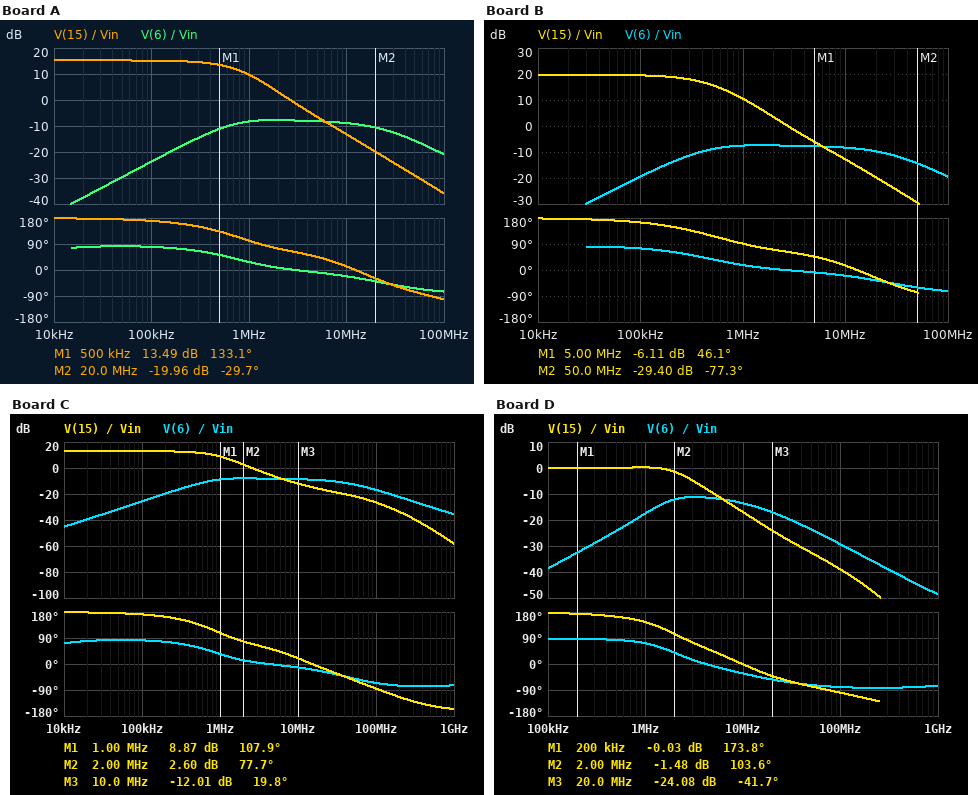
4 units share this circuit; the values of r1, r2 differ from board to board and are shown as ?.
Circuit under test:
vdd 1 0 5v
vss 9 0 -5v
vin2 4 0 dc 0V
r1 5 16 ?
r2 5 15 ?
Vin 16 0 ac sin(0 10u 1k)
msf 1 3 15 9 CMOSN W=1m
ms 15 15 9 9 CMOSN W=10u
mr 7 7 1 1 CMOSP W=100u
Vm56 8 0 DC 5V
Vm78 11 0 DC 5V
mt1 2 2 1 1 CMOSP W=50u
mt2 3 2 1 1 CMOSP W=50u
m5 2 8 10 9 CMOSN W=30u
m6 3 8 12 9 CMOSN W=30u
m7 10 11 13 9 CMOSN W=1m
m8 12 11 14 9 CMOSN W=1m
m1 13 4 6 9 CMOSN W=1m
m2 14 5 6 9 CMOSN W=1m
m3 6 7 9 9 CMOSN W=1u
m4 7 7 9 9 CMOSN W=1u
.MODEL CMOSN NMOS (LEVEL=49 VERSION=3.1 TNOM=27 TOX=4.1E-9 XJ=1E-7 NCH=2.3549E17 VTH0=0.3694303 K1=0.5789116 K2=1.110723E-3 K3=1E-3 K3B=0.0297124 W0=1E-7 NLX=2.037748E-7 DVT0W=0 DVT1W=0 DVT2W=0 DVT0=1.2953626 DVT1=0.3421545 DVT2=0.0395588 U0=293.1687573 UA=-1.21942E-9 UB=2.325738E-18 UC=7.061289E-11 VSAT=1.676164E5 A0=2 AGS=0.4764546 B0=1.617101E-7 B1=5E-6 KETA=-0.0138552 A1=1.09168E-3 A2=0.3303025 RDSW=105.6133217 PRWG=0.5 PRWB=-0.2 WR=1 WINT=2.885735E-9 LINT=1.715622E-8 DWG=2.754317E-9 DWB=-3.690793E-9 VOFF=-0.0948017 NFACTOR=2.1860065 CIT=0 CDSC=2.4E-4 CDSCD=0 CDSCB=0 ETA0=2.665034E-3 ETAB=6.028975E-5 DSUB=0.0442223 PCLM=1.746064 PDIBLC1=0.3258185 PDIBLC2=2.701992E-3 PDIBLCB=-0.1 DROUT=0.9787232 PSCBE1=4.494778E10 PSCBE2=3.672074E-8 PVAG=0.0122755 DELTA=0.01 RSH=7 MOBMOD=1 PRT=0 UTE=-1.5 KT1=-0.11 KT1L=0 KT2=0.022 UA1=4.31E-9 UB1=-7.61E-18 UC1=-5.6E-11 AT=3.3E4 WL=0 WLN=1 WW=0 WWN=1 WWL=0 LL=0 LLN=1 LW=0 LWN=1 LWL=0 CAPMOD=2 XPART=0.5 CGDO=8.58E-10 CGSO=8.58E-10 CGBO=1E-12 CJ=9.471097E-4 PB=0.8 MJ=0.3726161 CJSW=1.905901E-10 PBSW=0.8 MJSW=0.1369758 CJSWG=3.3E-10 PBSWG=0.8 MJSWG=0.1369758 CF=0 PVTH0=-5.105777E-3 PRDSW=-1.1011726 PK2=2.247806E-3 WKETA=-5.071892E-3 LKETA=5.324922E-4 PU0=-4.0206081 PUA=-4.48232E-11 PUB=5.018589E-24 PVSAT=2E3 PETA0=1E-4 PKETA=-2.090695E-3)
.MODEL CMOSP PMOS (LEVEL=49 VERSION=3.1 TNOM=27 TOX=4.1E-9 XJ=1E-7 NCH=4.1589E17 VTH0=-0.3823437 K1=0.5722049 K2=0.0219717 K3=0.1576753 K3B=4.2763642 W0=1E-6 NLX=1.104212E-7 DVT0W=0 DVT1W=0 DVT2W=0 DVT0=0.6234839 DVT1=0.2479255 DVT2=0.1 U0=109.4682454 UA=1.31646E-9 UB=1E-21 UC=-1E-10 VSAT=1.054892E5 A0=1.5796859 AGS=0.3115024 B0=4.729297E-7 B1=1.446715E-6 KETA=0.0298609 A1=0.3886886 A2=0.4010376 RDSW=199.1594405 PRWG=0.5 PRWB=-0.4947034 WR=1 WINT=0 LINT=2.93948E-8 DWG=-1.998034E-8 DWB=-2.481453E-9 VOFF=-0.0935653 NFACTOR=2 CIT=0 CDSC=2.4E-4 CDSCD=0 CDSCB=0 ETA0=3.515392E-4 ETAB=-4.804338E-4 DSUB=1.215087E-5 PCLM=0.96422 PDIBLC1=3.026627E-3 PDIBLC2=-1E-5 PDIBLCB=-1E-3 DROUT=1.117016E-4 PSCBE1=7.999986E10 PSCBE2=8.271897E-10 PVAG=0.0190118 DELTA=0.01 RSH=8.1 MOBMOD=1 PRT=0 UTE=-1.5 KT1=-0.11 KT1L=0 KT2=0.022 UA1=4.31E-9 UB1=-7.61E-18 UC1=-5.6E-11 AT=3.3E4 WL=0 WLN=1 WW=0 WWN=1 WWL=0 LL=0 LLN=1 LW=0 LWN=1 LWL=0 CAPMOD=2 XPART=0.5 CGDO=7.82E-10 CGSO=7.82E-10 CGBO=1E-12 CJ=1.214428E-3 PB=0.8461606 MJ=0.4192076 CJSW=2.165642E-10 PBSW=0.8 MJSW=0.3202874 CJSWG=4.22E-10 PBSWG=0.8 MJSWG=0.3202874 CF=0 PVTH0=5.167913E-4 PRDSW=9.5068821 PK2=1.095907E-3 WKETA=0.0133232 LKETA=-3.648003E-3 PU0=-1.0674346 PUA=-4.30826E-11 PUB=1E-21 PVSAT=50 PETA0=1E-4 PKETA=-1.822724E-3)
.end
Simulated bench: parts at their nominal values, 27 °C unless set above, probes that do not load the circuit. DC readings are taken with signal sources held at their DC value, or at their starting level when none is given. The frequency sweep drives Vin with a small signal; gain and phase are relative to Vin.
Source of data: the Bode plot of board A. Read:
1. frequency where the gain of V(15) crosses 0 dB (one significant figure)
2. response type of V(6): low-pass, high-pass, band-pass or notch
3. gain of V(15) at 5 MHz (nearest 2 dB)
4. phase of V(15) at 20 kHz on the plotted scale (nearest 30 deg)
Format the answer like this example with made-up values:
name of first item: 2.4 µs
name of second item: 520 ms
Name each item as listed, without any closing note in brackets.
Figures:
frequency where the gain of V(15) crosses 0 dB: 3 MHz
response type of V(6): low-pass, high-pass, band-pass or notch: band-pass
gain of V(15) at 5 MHz: -6 dB
phase of V(15) at 20 kHz on the plotted scale: 180 deg
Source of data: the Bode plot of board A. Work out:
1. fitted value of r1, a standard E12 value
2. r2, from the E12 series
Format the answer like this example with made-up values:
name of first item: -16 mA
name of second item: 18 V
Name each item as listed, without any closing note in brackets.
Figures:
fitted value of r1, a standard E12 value: 560 Ω
r2, from the E12 series: 3.3 kΩ
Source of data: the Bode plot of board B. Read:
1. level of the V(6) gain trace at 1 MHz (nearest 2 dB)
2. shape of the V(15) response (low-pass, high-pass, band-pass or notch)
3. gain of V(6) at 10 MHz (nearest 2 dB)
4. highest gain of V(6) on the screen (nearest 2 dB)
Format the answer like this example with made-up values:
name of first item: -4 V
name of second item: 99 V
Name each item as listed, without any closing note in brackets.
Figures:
level of the V(6) gain trace at 1 MHz: -8 dB
shape of the V(15) response: low-pass
gain of V(6) at 10 MHz: -8 dB
highest gain of V(6) on the screen: -8 dB
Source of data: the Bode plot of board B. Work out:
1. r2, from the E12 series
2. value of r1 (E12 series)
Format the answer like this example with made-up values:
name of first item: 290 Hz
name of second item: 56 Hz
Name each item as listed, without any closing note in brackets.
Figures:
r2, from the E12 series: 4.7 kΩ
value of r1: 470 Ω
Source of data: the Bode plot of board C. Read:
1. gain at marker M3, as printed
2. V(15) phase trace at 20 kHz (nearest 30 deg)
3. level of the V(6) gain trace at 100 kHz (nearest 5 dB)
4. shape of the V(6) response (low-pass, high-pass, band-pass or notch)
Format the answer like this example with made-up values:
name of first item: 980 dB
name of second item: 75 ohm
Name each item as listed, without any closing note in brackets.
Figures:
gain at marker M3, as printed: -12.01 dB
V(15) phase trace at 20 kHz: 180 deg
level of the V(6) gain trace at 100 kHz: -25 dB
shape of the V(6) response: band-pass
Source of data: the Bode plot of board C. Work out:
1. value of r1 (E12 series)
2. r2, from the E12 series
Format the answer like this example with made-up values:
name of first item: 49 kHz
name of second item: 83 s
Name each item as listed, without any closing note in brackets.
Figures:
value of r1: 330 Ω
r2, from the E12 series: 1.5 kΩ
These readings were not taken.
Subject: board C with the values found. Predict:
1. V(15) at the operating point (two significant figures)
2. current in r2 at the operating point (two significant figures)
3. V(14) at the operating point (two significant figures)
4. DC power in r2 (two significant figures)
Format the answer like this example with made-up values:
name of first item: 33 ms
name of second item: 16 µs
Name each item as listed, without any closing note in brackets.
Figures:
V(15) at the operating point: 26 mV
current in r2 at the operating point: 14 µA
V(14) at the operating point: 1.5 V
DC power in r2: 300 nW
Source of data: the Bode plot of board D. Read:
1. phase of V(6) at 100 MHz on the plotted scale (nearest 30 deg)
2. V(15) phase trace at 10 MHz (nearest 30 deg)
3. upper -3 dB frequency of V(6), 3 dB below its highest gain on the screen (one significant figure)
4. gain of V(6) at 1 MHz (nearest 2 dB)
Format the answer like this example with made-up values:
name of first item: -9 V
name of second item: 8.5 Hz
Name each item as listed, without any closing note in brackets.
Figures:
phase of V(6) at 100 MHz on the plotted scale: -90 deg
V(15) phase trace at 10 MHz: 0 deg
upper -3 dB frequency of V(6), 3 dB below its highest gain on the screen: 10 MHz
gain of V(6) at 1 MHz: -18 dB
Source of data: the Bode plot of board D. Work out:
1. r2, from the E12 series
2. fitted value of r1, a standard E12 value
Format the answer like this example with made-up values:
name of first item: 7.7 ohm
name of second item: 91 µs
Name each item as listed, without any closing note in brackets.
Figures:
r2, from the E12 series: 1.5 kΩ
fitted value of r1, a standard E12 value: 1.5 kΩ
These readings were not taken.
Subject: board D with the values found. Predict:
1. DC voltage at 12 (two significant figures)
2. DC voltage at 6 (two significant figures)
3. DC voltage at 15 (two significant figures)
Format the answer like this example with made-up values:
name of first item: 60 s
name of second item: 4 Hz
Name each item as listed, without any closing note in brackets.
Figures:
DC voltage at 12: 1.5 V
DC voltage at 6: -1.1 V
DC voltage at 15: 9.4 mV
